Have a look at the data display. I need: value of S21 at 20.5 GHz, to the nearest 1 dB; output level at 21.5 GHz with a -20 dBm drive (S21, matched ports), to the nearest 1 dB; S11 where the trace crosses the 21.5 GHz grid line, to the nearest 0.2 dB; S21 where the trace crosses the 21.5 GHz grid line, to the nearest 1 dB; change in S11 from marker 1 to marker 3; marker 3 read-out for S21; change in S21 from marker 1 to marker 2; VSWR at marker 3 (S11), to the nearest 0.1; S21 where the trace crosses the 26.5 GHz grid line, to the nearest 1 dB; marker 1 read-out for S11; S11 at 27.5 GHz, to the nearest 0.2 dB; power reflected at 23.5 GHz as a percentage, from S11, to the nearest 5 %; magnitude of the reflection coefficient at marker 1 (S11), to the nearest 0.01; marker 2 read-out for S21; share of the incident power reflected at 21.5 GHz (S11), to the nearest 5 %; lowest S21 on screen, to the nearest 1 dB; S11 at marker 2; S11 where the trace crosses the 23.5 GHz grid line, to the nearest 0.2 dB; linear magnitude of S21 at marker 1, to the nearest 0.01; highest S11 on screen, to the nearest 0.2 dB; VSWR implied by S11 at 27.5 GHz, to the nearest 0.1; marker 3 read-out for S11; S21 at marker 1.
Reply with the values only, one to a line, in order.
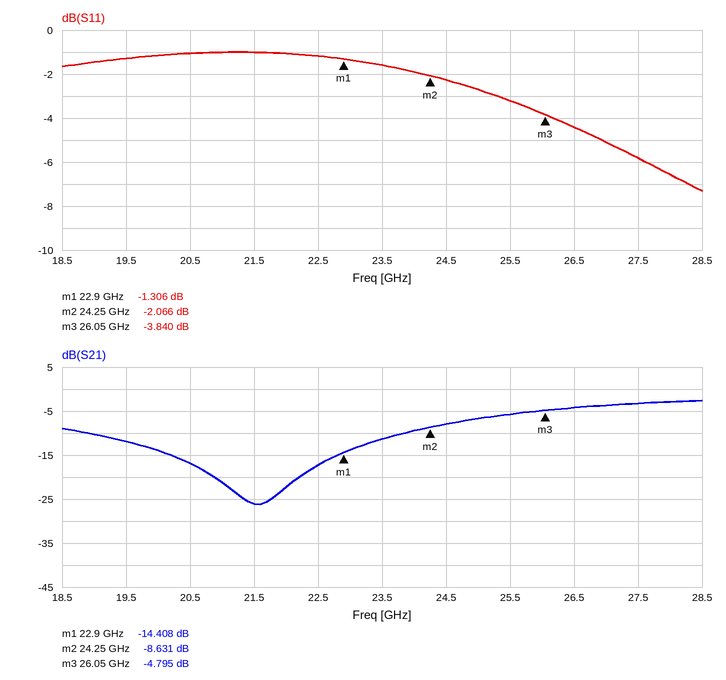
-17 dB
-46 dBm
-1.0 dB
-26 dB
-2.534 dB
-4.795 dB
5.777 dB
4.6
-4 dB
-1.306 dB
-5.8 dB
70 %
0.86
-8.631 dB
80 %
-26 dB
-2.066 dB
-1.6 dB
0.19
-1.0 dB
3.1
-3.840 dB
-14.408 dB
